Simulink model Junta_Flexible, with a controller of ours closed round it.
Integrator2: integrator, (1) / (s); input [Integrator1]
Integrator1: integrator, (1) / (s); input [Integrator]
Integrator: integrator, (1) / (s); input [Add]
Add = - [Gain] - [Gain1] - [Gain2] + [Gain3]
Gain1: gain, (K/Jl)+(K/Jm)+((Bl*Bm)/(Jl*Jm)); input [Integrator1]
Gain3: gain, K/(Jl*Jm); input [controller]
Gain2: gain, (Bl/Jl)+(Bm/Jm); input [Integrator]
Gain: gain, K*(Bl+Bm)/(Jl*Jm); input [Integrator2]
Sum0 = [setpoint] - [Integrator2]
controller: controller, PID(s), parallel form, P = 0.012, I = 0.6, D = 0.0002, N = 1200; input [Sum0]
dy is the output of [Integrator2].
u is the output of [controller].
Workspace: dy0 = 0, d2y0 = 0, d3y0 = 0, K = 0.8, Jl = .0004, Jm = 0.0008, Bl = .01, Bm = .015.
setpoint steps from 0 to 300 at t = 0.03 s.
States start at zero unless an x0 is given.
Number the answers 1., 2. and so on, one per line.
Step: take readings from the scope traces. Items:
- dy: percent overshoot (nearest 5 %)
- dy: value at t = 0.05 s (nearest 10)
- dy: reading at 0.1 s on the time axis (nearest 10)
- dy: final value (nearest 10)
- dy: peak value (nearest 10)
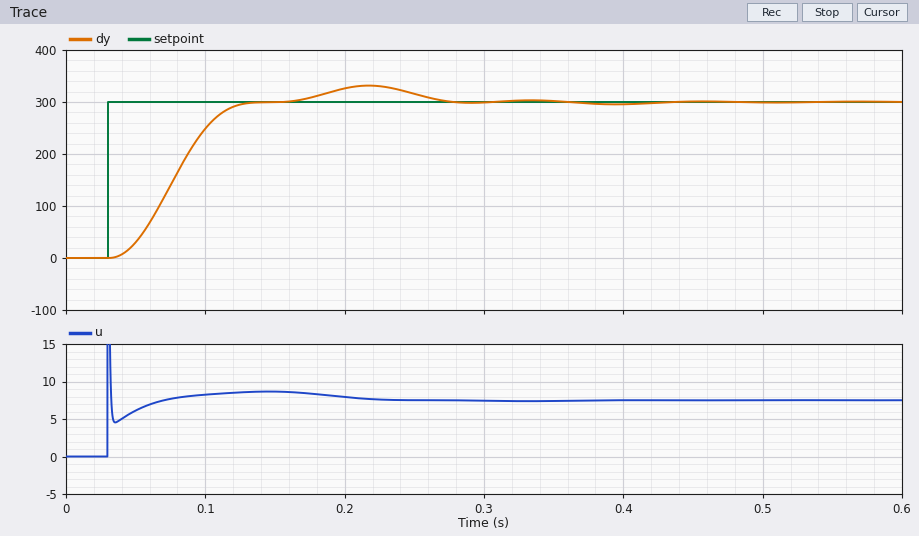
1. 10 %
2. 30
3. 250
4. 300
5. 330
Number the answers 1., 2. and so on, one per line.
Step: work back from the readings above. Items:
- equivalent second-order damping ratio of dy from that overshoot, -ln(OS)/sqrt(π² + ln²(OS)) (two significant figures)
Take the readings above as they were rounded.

1. 0.59
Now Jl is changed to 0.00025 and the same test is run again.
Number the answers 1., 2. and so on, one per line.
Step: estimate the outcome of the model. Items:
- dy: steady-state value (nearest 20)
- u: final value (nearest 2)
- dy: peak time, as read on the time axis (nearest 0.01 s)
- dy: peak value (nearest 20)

1. 300
2. 8
3. 0.19 s
4. 320
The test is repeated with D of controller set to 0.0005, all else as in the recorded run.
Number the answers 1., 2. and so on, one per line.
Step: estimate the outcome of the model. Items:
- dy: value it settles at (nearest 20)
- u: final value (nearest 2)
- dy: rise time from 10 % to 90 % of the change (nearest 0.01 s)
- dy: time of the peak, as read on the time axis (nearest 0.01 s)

1. 300
2. 8
3. 0.10 s
4. 0.19 s
